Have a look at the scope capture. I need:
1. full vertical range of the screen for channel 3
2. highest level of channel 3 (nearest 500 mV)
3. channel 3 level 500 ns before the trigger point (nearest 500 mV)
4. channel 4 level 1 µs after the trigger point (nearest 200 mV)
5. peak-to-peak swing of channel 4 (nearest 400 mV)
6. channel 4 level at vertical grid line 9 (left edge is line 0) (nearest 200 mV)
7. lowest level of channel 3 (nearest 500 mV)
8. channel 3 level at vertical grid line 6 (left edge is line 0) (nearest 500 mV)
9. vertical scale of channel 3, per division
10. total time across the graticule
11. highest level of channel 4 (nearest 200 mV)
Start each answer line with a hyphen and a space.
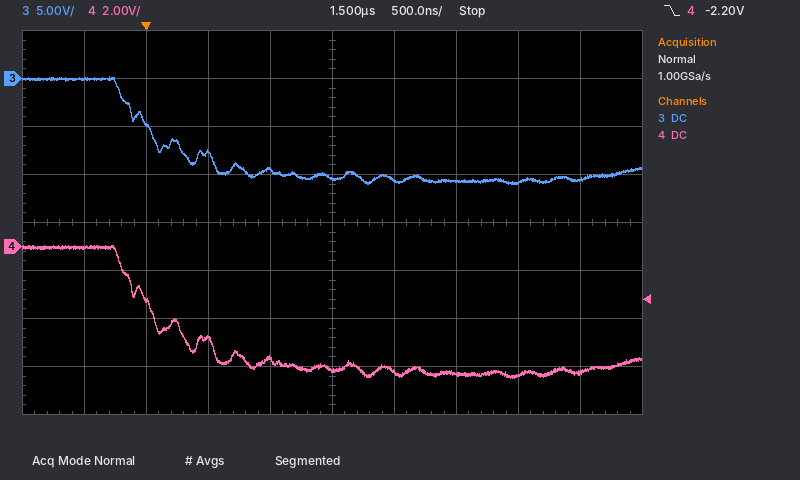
- 40 V
- 0.0 V
- 0.0 V
- -4.8 V
- 5.6 V
- -5.2 V
- -11.0 V
- -10.5 V
- 5 V
- 5 µs
- 0.0 V
